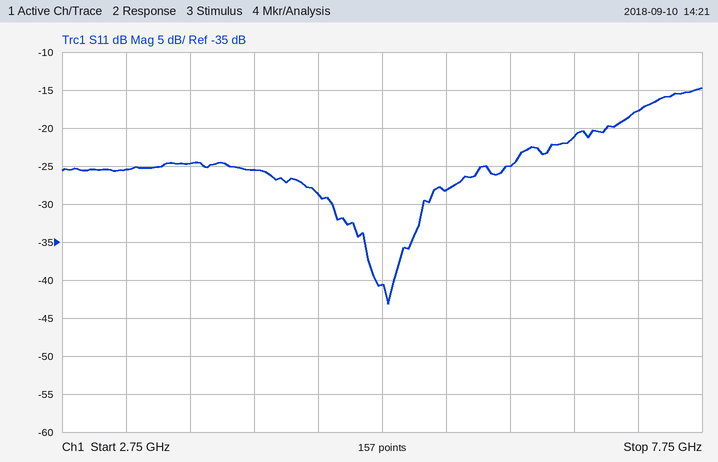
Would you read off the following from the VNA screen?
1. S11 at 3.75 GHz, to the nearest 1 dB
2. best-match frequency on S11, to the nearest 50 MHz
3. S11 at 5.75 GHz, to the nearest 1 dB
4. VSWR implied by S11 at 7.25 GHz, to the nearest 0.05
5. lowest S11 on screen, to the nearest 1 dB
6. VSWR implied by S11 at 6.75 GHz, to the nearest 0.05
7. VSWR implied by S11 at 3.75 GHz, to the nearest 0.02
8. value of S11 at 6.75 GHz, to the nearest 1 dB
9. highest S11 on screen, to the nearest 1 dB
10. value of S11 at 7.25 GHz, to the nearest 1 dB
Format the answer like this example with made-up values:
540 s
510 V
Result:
-25 dB
5.30 GHz
-28 dB
1.30
-43 dB
1.20
1.12
-21 dB
-15 dB
-18 dB
